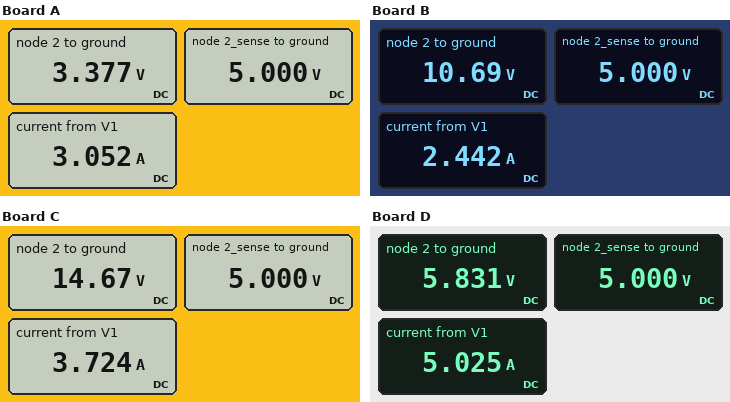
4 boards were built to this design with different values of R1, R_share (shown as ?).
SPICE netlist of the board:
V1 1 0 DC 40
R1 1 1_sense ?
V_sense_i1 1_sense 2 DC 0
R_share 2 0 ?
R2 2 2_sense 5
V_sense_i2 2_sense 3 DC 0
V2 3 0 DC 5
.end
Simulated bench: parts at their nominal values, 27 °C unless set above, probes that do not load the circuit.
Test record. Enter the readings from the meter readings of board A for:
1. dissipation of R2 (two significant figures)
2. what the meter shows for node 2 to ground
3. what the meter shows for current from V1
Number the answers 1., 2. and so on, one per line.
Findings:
1. 530 mW
2. 3.377 V
3. 3.052 A
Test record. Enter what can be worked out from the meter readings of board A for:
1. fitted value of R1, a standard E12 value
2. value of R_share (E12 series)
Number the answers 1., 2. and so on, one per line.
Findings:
1. 12 Ω
2. 1 Ω
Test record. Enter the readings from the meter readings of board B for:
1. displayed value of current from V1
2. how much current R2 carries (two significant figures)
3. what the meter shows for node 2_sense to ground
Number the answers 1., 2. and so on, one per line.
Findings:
1. 2.442 A
2. 1.1 A
3. 5.000 V
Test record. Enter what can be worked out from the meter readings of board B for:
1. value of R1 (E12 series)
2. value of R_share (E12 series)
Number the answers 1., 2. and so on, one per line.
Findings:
1. 12 Ω
2. 8.2 Ω
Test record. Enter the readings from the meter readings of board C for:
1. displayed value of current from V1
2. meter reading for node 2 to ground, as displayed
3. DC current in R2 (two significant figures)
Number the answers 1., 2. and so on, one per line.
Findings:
1. 3.724 A
2. 14.67 V
3. 1.9 A
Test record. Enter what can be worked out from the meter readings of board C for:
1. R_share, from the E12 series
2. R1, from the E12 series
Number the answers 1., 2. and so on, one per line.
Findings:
1. 8.2 Ω
2. 6.8 Ω
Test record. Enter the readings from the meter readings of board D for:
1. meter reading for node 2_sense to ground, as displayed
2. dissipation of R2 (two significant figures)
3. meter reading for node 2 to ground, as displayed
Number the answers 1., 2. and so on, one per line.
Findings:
1. 5.000 V
2. 140 mW
3. 5.831 V
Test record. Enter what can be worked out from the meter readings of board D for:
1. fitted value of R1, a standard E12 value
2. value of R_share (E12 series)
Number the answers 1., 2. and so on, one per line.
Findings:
1. 6.8 Ω
2. 1.2 Ω
